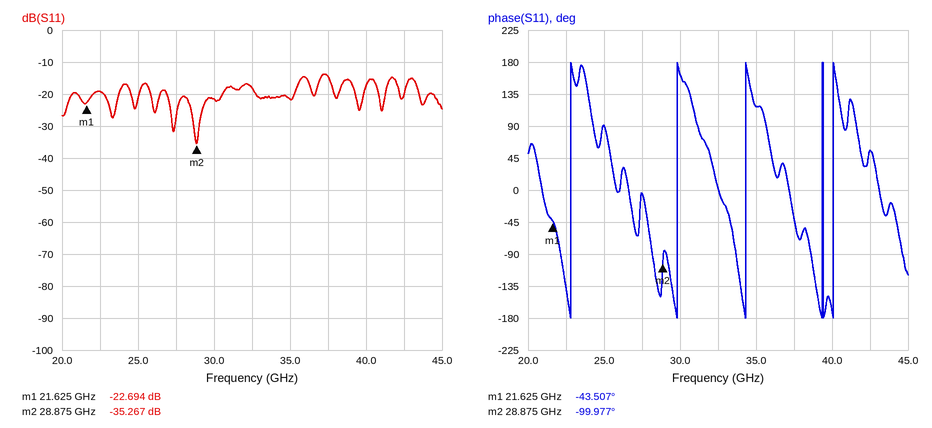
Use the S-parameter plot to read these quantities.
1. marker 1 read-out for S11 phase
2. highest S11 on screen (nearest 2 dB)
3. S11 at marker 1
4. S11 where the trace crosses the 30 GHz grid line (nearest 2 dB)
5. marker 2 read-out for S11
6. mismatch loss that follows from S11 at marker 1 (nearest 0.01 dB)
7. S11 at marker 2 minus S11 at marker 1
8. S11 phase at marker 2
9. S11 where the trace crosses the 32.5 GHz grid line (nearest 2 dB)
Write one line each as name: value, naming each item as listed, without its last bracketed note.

marker 1 read-out for S11 phase: -43.507°
highest S11 on screen: -14 dB
S11 at marker 1: -22.694 dB
S11 where the trace crosses the 30 GHz grid line: -22 dB
marker 2 read-out for S11: -35.267 dB
mismatch loss that follows from S11 at marker 1: 0.02 dB
S11 at marker 2 minus S11 at marker 1: -12.573 dB
S11 phase at marker 2: -99.977°
S11 where the trace crosses the 32.5 GHz grid line: -18 dB
